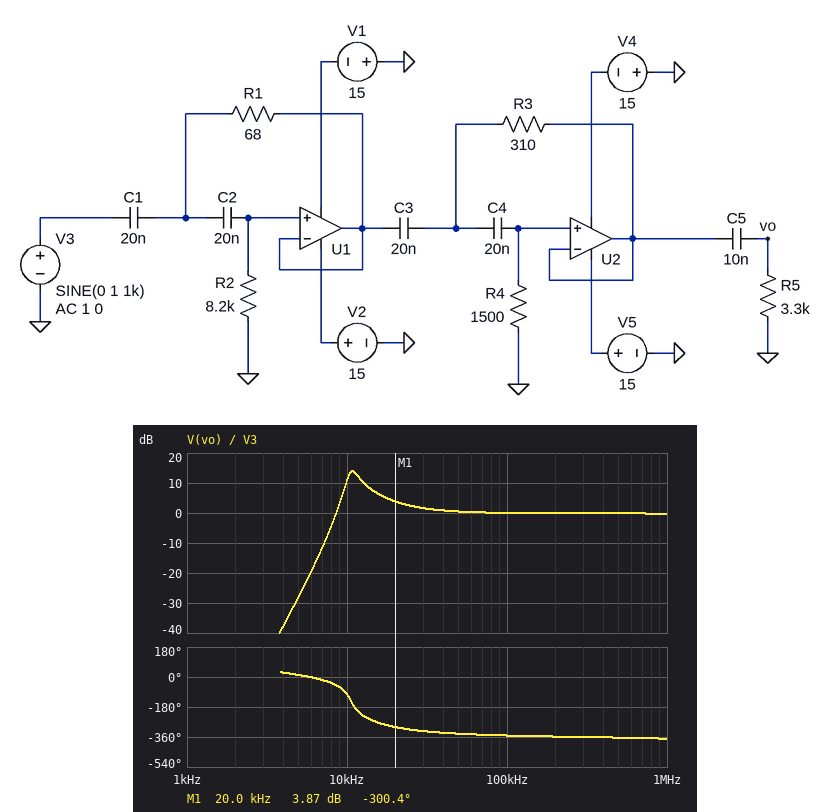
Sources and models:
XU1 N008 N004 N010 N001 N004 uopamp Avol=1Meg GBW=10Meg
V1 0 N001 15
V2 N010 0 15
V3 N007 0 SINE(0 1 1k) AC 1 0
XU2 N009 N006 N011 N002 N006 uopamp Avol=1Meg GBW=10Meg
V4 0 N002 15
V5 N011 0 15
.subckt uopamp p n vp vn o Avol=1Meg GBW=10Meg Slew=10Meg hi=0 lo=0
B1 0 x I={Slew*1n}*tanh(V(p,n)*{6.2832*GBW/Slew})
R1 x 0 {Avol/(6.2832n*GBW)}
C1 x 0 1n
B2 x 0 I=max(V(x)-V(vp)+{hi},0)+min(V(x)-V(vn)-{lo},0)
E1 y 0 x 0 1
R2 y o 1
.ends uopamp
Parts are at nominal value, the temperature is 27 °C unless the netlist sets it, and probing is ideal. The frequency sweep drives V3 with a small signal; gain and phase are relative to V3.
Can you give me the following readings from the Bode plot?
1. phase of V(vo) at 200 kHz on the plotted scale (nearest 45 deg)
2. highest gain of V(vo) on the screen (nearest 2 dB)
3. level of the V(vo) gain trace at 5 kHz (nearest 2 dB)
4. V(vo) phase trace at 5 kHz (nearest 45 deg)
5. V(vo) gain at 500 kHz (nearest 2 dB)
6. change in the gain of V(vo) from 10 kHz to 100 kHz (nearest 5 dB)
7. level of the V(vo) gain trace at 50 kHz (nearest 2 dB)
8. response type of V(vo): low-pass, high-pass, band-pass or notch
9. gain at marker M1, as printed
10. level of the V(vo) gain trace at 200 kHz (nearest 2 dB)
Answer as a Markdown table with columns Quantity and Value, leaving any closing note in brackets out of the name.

| Quantity | Value |
|---|---|
| phase of V(vo) at 200 kHz on the plotted scale | -360 deg |
| highest gain of V(vo) on the screen | 14 dB |
| level of the V(vo) gain trace at 5 kHz | -28 dB |
| V(vo) phase trace at 5 kHz | 0 deg |
| V(vo) gain at 500 kHz | 0 dB |
| change in the gain of V(vo) from 10 kHz to 100 kHz | -10 dB |
| level of the V(vo) gain trace at 50 kHz | 0 dB |
| response type of V(vo): low-pass, high-pass, band-pass or notch | high-pass |
| gain at marker M1, as printed | 3.87 dB |
| level of the V(vo) gain trace at 200 kHz | 0 dB |
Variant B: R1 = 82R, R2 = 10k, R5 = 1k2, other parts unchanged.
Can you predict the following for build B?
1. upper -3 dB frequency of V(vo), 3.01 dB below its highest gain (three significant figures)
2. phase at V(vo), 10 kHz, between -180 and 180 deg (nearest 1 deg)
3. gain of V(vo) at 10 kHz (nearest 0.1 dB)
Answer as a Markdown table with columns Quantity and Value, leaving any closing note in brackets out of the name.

| Quantity | Value |
|---|---|
| upper -3 dB frequency of V(vo), 3.01 dB below its highest gain | 11.6 kHz |
| phase at V(vo), 10 kHz, between -180 and 180 deg | -165 deg |
| gain of V(vo) at 10 kHz | 5.5 dB |
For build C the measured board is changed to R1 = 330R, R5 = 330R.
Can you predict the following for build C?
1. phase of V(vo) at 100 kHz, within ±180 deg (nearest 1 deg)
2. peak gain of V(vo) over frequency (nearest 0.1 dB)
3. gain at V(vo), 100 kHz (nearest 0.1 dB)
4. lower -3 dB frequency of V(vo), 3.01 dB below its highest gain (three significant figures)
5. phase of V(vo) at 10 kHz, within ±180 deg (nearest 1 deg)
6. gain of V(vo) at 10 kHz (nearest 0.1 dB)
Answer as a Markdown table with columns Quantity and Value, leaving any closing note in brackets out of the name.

| Quantity | Value |
|---|---|
| phase of V(vo) at 100 kHz, within ±180 deg | 32 deg |
| peak gain of V(vo) over frequency | -0.1 dB |
| gain at V(vo), 100 kHz | -0.9 dB |
| lower -3 dB frequency of V(vo), 3.01 dB below its highest gain | 43.0 kHz |
| phase of V(vo) at 10 kHz, within ±180 deg | -159 deg |
| gain of V(vo) at 10 kHz | -12.8 dB |
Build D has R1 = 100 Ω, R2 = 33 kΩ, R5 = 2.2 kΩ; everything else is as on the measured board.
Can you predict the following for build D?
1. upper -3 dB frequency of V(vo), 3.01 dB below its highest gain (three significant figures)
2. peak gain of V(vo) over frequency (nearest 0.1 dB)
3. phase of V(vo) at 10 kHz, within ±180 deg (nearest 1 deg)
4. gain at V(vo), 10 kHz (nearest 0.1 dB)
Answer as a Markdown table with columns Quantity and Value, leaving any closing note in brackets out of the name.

| Quantity | Value |
|---|---|
| upper -3 dB frequency of V(vo), 3.01 dB below its highest gain | 4.04 MHz |
| peak gain of V(vo) over frequency | 1.6 dB |
| phase of V(vo) at 10 kHz, within ±180 deg | 148 deg |
| gain at V(vo), 10 kHz | -1.1 dB |
